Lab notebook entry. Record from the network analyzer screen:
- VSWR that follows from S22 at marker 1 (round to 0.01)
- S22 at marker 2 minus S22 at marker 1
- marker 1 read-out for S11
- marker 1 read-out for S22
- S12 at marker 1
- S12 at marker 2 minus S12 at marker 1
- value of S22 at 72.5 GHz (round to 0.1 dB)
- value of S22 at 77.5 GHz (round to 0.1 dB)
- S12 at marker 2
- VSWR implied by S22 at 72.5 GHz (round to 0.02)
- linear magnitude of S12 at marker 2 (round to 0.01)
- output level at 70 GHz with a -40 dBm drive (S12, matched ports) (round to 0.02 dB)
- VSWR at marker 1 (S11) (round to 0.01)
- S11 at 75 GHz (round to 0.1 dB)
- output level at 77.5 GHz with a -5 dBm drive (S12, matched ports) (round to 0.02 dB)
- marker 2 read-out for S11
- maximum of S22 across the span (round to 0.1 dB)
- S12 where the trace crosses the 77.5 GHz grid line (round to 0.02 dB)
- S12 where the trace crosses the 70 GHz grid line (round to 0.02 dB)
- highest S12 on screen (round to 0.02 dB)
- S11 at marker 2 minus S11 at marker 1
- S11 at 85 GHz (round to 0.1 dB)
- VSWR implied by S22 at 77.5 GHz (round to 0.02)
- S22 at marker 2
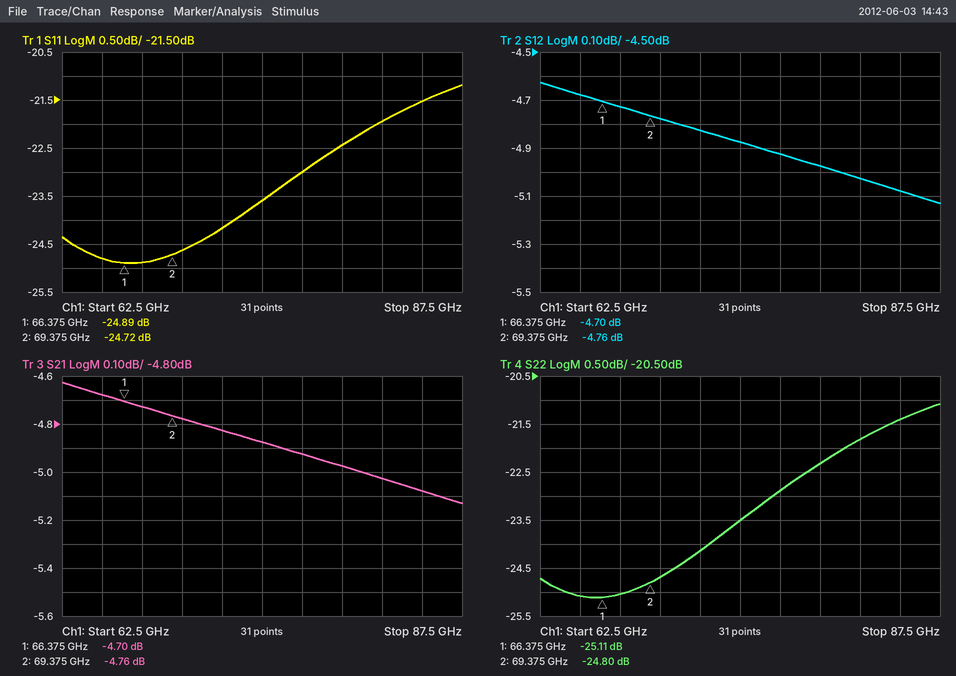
1.12
0.31 dB
-24.89 dB
-25.11 dB
-4.70 dB
-0.06 dB
-24.1 dB
-22.9 dB
-4.76 dB
1.14
0.58
-44.78 dBm
1.12
-23.6 dB
-9.92 dBm
-24.72 dB
-21.1 dB
-4.92 dB
-4.78 dB
-4.62 dB
0.17 dB
-21.5 dB
1.16
-24.80 dB
